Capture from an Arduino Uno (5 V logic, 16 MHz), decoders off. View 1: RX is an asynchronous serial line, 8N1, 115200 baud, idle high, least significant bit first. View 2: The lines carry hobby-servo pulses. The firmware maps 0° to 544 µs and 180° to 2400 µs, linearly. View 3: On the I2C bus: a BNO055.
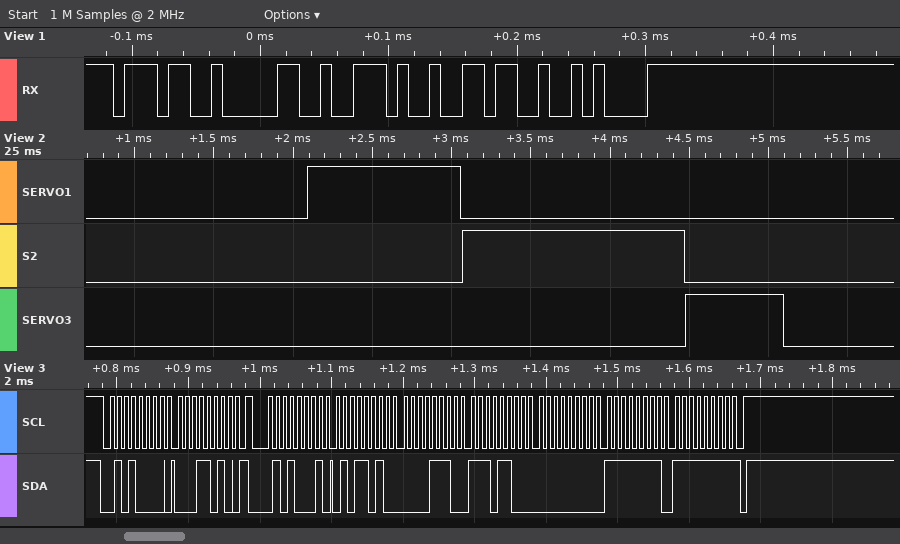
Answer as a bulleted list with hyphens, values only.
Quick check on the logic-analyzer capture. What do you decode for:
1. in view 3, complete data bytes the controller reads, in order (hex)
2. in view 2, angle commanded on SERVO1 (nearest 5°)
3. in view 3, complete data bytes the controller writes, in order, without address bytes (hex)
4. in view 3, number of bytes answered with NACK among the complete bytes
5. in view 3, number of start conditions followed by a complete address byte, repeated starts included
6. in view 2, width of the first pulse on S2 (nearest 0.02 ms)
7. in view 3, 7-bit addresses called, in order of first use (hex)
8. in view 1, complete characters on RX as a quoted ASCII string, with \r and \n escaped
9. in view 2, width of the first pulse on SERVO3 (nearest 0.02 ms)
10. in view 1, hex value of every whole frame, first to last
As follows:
- 5A 0E EC 00 FF FF
- 40°
- 1A
- 1
- 2
- 1.40 ms
- 0x28
- "70.6\n"
- 0.62 ms
- 37 30 2E 36 0A
